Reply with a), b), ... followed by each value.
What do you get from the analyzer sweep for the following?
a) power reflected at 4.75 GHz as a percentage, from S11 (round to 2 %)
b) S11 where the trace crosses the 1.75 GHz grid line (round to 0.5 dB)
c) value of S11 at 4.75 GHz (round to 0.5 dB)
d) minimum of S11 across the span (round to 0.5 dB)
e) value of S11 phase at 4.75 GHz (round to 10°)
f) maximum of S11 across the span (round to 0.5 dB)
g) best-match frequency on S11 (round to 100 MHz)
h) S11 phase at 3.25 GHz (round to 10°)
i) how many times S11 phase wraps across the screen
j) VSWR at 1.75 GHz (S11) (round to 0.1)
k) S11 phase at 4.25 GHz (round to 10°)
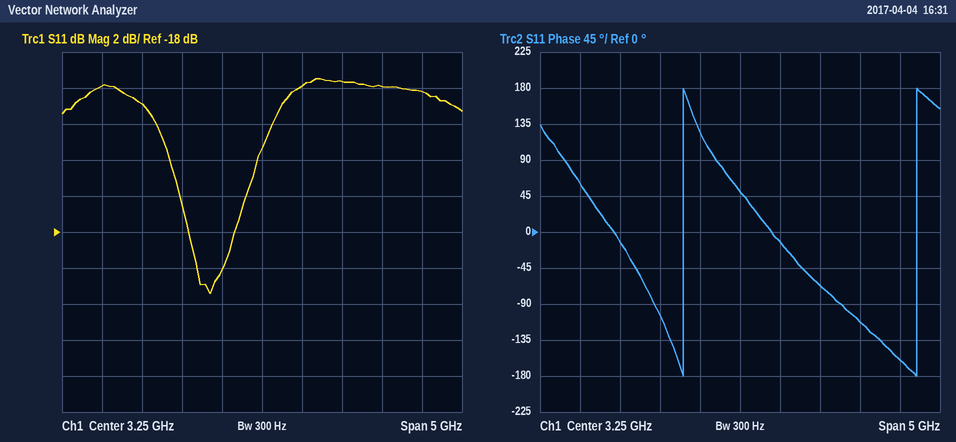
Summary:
a) 10 %
b) -11.0 dB
c) -10.0 dB
d) -21.5 dB
e) -110°
f) -9.5 dB
g) 2.6 GHz
h) 50°
i) 2
j) 1.8
k) -70°
